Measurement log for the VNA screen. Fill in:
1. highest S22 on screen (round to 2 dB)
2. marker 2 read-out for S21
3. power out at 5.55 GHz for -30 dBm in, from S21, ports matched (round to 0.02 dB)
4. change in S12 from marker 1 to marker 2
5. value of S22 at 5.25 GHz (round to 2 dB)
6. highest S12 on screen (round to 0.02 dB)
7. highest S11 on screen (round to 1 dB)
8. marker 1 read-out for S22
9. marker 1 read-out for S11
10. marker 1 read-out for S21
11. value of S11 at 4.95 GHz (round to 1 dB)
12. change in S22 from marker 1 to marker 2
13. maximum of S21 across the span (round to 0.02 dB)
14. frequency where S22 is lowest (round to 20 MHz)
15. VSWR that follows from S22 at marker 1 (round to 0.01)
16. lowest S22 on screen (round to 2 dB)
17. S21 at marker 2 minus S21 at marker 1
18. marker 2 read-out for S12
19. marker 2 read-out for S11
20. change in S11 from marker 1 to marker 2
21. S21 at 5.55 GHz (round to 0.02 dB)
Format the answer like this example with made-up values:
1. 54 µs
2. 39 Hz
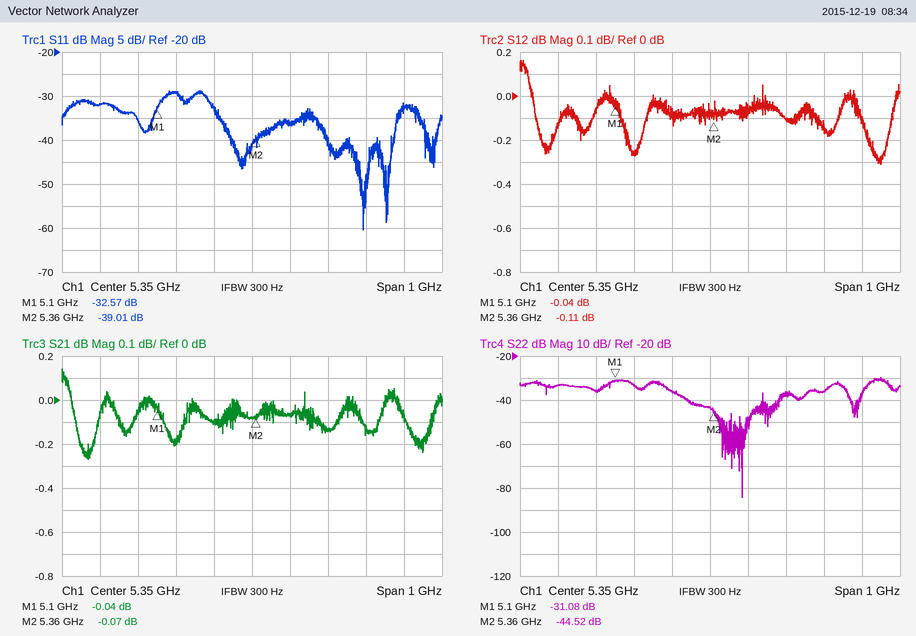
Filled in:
1. -30 dB
2. -0.07 dB
3. -30.14 dBm
4. -0.07 dB
5. -36 dB
6. 0.16 dB
7. -29 dB
8. -31.08 dB
9. -32.57 dB
10. -0.04 dB
11. -32 dB
12. -13.44 dB
13. 0.14 dB
14. 5.44 GHz
15. 1.06
16. -84 dB
17. -0.03 dB
18. -0.11 dB
19. -39.01 dB
20. -6.44 dB
21. -0.14 dB
